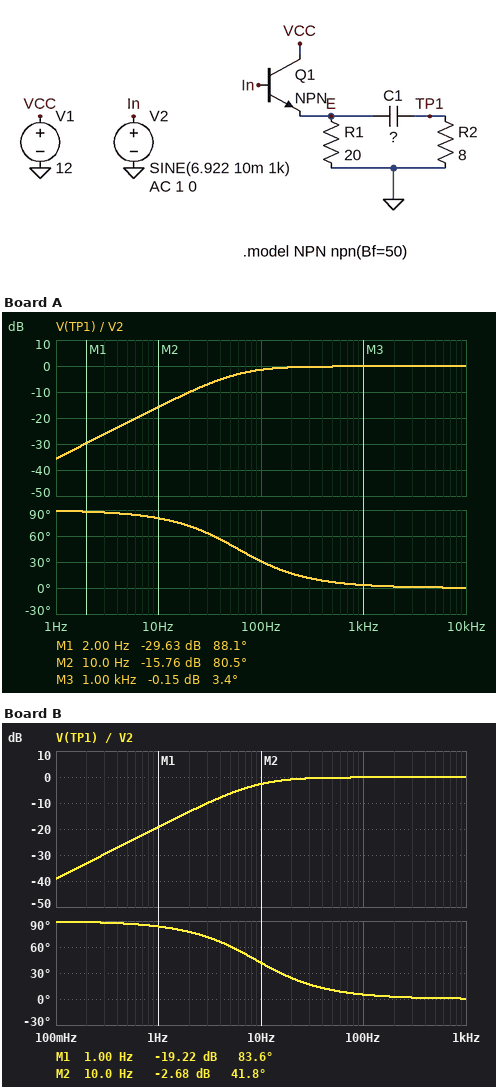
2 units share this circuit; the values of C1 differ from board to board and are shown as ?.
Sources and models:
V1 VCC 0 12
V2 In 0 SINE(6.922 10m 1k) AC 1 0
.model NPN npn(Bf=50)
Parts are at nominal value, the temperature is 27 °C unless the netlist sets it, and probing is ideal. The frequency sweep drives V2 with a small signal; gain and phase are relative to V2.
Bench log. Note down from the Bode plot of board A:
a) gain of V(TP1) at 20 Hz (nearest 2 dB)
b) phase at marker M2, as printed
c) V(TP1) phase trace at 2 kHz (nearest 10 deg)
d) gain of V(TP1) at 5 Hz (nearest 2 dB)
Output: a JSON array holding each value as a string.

["-10 dB", "80.5 deg", "0 deg", "-22 dB"]
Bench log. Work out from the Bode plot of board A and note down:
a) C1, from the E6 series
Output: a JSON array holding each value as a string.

["330 µF"]
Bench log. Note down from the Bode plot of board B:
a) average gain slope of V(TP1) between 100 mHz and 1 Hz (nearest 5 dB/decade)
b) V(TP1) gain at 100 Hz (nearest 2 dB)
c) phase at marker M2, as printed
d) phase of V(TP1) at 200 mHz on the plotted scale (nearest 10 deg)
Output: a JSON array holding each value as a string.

["20 dB/decade", "0 dB", "41.8 deg", "90 deg"]
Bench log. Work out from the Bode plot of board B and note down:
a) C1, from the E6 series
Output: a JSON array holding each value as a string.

["2.2 mF"]
